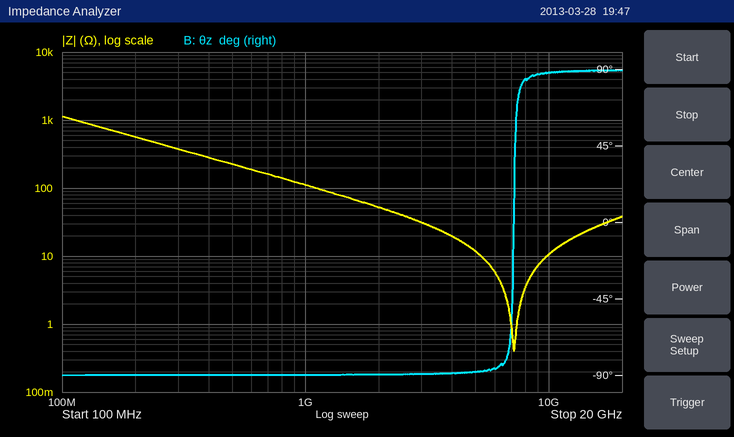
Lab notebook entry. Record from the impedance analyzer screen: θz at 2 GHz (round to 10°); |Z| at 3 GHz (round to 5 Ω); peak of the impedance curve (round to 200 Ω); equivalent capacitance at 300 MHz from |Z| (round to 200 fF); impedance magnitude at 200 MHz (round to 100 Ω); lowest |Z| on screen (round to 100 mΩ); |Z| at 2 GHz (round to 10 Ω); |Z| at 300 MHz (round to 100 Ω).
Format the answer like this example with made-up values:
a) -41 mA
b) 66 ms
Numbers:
a) -90°
b) 30 Ω
c) 1.2 kΩ
d) 1.4 pF
e) 600 Ω
f) 400 mΩ
g) 50 Ω
h) 400 Ω
